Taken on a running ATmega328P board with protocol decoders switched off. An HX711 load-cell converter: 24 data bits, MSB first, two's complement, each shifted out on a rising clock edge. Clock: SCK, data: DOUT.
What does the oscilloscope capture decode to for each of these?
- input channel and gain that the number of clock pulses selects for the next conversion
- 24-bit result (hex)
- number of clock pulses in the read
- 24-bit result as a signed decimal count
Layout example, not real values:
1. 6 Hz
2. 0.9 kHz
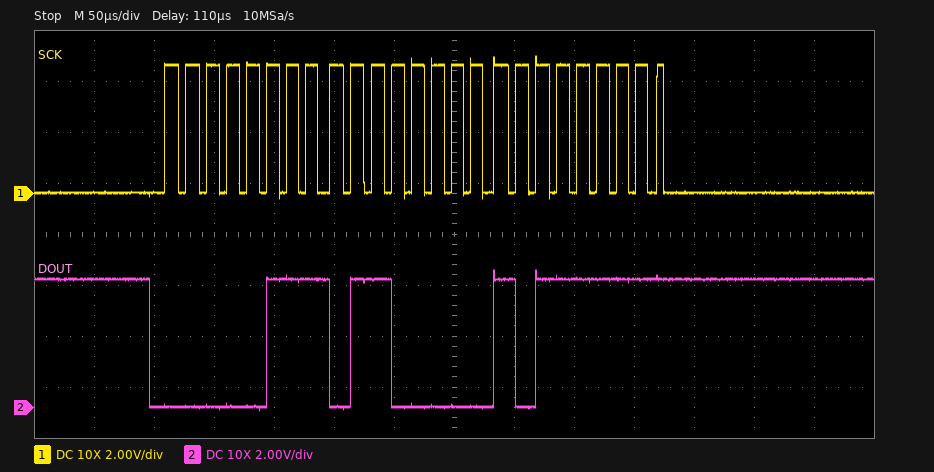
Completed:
1. channel A, gain 128
2. 0x0760BF
3. 25
4. 483519
